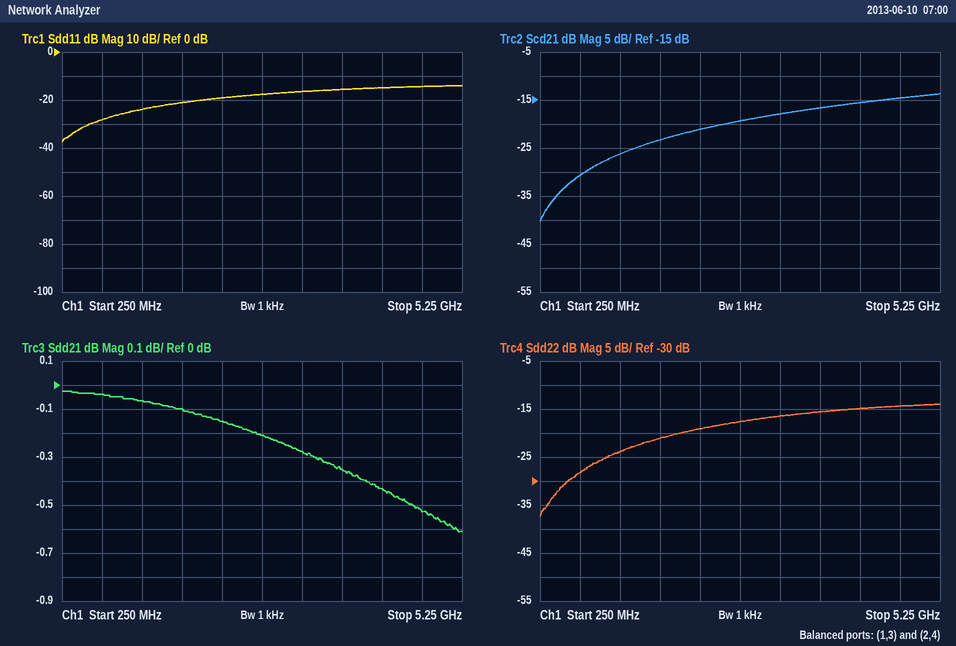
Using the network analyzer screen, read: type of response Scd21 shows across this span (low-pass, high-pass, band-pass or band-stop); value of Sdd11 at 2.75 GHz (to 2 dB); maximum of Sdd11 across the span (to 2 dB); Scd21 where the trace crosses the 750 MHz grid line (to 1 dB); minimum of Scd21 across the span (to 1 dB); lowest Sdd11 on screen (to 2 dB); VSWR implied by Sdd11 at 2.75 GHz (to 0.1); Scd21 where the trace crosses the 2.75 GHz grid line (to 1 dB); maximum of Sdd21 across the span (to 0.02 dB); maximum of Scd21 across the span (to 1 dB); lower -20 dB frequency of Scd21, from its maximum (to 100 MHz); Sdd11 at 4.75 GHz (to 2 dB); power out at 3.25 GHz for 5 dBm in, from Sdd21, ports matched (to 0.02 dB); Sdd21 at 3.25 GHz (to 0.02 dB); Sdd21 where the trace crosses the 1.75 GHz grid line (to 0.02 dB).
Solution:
high-pass
-18 dB
-14 dB
-31 dB
-40 dB
-38 dB
1.3
-19 dB
-0.02 dB
-14 dB
500 MHz
-14 dB
4.72 dBm
-0.28 dB
-0.10 dB
